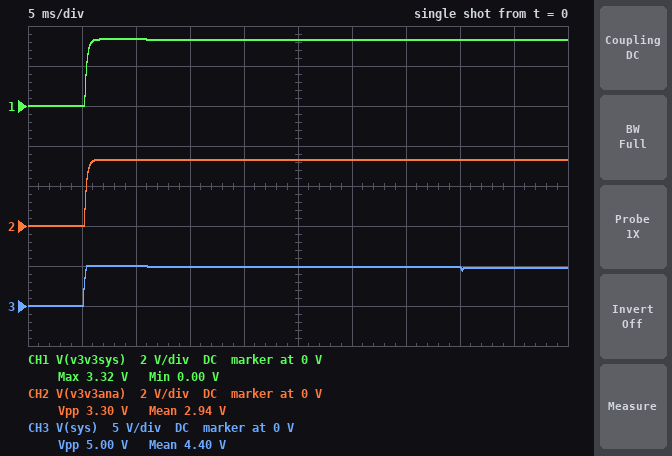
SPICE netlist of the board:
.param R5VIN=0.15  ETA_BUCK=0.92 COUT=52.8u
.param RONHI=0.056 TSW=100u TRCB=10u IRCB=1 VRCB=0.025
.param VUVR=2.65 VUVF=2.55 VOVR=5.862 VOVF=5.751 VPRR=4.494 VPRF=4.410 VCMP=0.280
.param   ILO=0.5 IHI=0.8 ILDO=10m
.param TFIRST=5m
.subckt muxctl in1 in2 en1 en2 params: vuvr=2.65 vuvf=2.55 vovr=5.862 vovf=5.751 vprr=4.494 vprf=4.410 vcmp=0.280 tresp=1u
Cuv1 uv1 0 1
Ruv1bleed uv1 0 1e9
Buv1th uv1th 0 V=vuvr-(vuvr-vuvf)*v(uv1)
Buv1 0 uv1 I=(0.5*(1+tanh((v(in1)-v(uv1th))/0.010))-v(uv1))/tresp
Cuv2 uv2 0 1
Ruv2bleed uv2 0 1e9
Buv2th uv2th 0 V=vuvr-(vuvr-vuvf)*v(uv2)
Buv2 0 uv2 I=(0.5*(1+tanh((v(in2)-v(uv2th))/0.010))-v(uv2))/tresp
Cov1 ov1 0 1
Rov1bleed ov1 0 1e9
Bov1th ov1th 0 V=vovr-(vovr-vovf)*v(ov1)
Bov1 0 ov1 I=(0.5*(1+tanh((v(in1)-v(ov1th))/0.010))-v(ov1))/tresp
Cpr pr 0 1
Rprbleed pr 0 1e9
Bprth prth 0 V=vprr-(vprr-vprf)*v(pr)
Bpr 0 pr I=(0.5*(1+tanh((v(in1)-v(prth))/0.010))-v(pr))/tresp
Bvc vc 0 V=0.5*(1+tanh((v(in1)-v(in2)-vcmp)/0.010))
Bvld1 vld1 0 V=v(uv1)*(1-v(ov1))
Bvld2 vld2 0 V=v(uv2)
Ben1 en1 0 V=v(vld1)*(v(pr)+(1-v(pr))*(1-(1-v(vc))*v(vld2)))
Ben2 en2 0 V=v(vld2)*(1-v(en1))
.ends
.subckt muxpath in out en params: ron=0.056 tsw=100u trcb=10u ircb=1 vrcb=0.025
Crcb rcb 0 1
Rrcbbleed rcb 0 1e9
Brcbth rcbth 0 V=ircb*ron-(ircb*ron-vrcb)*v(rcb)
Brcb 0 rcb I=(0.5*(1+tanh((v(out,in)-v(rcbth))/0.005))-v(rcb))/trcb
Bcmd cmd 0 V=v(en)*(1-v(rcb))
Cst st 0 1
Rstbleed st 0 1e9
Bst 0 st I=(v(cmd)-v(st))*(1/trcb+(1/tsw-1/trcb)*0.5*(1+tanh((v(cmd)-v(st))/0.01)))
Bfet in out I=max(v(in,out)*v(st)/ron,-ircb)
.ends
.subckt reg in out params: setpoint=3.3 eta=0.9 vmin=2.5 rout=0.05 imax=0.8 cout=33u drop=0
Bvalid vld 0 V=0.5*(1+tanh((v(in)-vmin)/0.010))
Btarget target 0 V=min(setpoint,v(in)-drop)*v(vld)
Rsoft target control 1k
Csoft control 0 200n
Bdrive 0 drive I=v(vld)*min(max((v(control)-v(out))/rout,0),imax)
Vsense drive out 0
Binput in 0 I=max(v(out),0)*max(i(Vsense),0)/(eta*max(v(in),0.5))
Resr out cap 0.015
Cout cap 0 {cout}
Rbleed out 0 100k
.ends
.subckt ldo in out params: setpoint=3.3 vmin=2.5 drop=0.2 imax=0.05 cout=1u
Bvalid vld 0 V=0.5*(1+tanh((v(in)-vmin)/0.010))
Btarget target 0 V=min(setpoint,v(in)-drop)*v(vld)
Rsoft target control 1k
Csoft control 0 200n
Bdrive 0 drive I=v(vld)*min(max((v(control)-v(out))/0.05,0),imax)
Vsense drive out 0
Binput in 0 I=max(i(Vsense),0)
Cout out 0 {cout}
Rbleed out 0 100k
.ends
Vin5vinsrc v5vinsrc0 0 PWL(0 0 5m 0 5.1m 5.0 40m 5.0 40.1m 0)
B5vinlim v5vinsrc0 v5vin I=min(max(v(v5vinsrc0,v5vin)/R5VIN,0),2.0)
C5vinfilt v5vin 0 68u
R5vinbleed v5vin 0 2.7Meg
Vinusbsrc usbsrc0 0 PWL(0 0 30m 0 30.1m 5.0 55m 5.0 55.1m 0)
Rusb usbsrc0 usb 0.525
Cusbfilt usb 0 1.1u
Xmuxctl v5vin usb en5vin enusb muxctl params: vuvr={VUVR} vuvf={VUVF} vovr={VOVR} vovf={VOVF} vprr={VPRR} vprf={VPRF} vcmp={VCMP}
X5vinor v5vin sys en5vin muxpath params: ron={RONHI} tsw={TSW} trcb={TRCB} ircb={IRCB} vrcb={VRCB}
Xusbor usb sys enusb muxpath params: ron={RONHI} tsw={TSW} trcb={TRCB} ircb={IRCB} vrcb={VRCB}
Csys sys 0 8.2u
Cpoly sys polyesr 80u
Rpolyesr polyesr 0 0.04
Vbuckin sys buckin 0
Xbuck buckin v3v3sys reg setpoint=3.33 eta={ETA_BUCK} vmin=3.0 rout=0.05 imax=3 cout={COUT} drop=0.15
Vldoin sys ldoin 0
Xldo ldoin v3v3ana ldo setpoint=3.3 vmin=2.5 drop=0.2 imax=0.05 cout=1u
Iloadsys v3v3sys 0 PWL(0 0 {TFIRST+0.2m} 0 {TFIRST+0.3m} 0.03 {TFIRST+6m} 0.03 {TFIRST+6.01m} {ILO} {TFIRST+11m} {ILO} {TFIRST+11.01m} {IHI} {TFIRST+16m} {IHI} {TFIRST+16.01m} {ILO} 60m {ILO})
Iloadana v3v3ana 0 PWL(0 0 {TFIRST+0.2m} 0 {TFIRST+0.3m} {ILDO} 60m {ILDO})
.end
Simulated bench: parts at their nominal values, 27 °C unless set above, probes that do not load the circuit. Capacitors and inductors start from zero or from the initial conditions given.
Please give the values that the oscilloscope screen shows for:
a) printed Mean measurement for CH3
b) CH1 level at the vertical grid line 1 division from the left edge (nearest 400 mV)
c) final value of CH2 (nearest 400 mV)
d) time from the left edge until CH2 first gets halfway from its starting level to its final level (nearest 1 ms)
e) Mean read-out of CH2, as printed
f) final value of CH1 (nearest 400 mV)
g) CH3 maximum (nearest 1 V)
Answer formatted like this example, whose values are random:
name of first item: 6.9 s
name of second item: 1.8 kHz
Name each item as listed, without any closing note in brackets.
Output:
printed Mean measurement for CH3: 4.40 V
CH1 level at the vertical grid line 1 division from the left edge: 0 V
final value of CH2: 3.2 V
time from the left edge until CH2 first gets halfway from its starting level to its final level: 5 ms
Mean read-out of CH2, as printed: 2.94 V
final value of CH1: 3.2 V
CH3 maximum: 5 V
